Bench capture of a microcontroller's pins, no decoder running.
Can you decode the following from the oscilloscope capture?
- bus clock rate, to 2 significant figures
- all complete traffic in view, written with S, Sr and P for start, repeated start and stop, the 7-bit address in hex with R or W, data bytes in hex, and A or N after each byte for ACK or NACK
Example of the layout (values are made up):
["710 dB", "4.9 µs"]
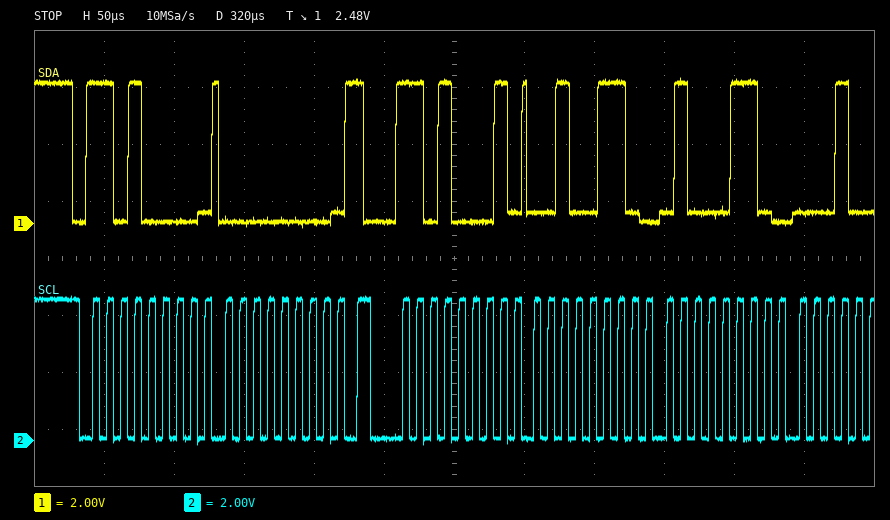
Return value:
["100 kHz", "S 68W A 00 A Sr 68R A 26 A 46 A"]
